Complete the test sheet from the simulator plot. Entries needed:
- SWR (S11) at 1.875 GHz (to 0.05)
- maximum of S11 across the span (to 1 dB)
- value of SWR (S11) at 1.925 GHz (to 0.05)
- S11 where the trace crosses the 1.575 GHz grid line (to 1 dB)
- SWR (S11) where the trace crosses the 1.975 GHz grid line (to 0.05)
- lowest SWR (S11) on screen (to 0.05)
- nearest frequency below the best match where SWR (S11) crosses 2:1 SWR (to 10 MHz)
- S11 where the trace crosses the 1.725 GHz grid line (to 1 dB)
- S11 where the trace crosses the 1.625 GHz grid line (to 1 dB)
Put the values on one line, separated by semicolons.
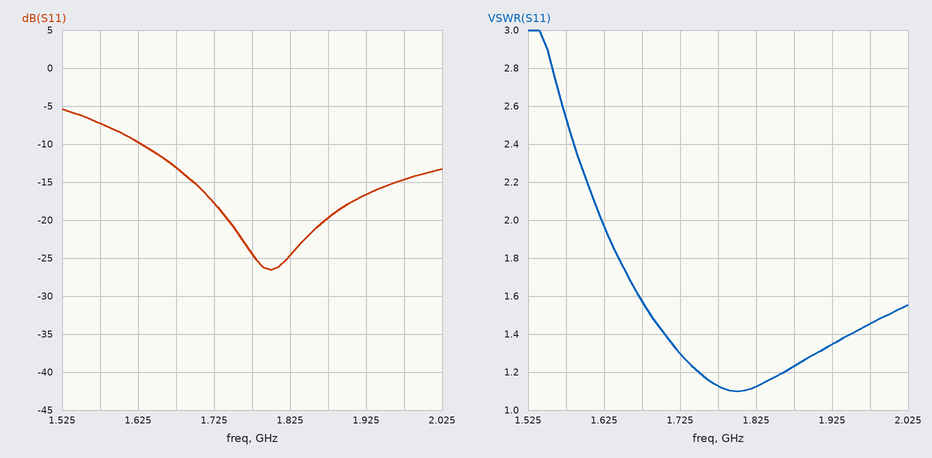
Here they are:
1.25; -5 dB; 1.35; -7 dB; 1.45; 1.10; 1.62 GHz; -18 dB; -10 dB
